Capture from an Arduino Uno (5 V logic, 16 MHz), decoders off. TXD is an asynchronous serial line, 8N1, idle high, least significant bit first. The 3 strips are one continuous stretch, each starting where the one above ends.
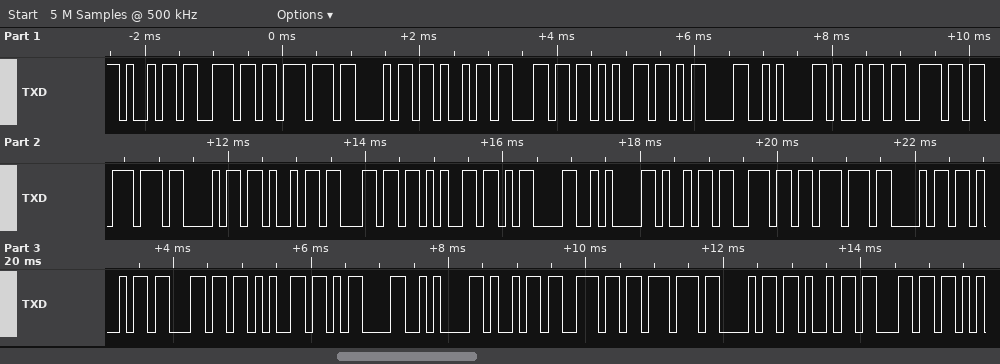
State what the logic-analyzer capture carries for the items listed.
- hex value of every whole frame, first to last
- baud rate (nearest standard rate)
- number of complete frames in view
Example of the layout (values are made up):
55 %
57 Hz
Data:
69 6E 77 68 69 6C 65 0D 0A 69 6E 77 68 69 6C 65 0D 0A 69 6E 77 68 69 6C 65 0D 0A 69 6E 77 68 69 6C
9600 baud
33
